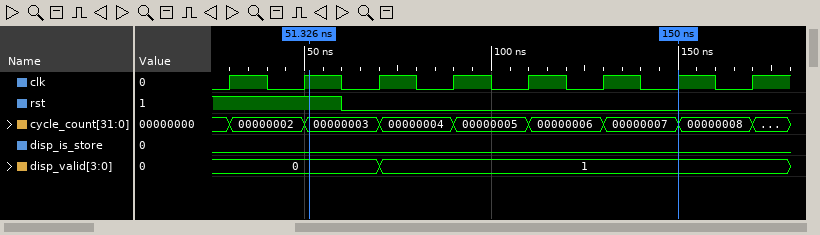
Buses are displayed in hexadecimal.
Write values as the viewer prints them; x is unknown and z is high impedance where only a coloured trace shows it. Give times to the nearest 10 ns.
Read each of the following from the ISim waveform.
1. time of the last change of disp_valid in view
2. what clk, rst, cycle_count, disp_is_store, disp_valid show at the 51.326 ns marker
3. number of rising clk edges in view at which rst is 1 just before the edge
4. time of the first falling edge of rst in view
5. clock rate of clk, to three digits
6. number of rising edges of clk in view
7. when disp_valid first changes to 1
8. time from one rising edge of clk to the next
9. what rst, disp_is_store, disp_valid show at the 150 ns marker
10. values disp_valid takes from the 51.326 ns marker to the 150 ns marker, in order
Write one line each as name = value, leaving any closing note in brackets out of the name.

time of the last change of disp_valid in view = 70 ns
what clk, rst, cycle_count, disp_is_store, disp_valid show at the 51.326 ns marker = clk=1, rst=1, cycle_count=00000003, disp_is_store=0, disp_valid=0
number of rising clk edges in view at which rst is 1 just before the edge = 2
time of the first falling edge of rst in view = 60 ns
clock rate of clk, to three digits = 50.0 MHz
number of rising edges of clk in view = 8
when disp_valid first changes to 1 = 70 ns
time from one rising edge of clk to the next = 20 ns
what rst, disp_is_store, disp_valid show at the 150 ns marker = rst=0, disp_is_store=0, disp_valid=1
values disp_valid takes from the 51.326 ns marker to the 150 ns marker, in order = 0, 1
